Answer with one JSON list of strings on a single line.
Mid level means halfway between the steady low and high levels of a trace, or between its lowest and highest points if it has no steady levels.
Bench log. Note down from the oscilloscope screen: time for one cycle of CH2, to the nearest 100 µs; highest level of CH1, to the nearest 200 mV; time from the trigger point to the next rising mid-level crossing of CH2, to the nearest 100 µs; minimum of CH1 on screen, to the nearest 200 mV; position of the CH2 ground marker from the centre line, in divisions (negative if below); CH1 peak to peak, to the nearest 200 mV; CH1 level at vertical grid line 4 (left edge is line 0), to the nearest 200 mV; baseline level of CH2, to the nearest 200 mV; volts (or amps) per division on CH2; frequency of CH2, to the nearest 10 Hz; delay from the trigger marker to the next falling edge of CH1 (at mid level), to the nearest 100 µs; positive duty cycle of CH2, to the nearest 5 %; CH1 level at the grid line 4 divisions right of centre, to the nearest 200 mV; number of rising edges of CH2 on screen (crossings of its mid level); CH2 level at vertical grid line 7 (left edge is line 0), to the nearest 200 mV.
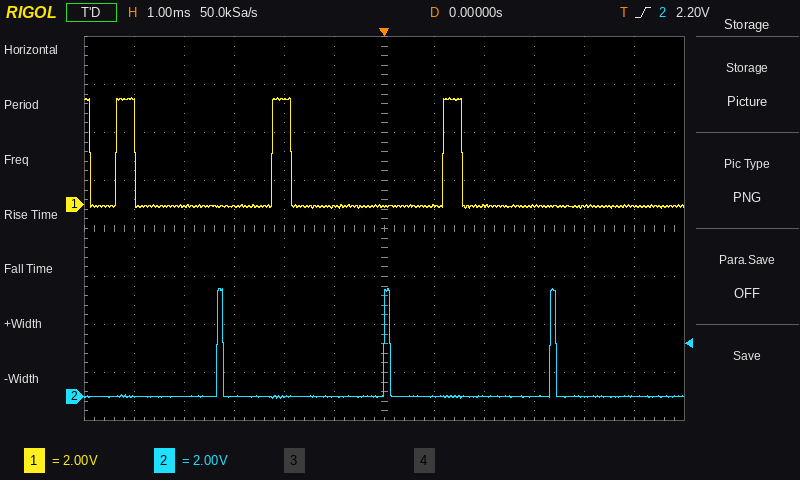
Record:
["3.3 ms", "4.4 V", "3.3 ms", "-200 mV", "-3.5 div", "4.6 V", "4.4 V", "0.0 V", "2 V", "300 Hz", "1.6 ms", "5 %", "0.0 V", "3", "0.0 V"]
